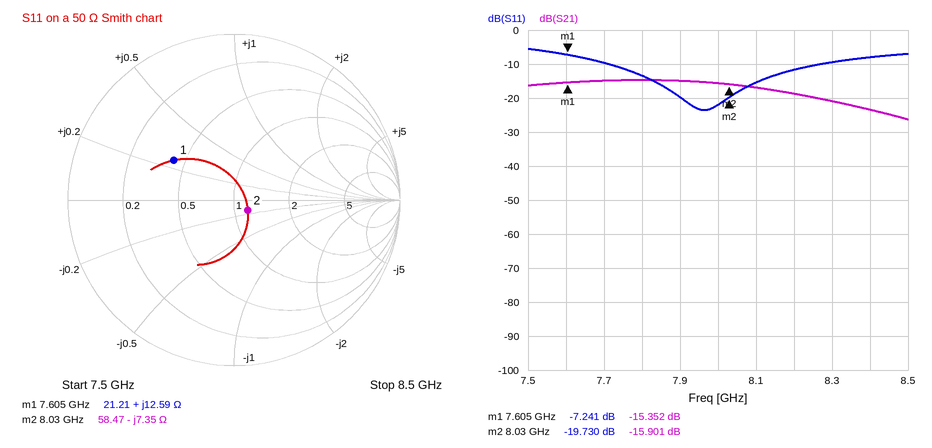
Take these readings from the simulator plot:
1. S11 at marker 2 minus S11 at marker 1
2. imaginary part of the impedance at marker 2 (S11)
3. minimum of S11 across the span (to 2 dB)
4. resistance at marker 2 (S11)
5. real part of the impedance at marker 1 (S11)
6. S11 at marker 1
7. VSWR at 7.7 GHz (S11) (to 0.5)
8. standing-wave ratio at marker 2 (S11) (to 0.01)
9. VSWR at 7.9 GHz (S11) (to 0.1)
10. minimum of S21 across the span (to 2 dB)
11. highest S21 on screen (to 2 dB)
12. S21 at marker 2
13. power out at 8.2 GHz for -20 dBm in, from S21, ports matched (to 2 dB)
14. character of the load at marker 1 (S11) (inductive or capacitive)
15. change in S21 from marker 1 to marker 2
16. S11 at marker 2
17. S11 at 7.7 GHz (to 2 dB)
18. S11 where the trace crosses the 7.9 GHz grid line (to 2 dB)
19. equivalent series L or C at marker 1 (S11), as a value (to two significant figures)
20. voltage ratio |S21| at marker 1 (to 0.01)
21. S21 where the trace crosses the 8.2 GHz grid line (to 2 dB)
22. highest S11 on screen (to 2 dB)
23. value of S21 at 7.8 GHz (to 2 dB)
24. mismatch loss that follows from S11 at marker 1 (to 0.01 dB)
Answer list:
-12.489 dB
-7.35 Ω
-24 dB
58.47 Ω
21.21 Ω
-7.241 dB
2.0
1.23
1.2
-26 dB
-14 dB
-15.901 dB
-38 dBm
inductive
-0.549 dB
-19.730 dB
-10 dB
-20 dB
260 pH
0.17
-18 dB
-6 dB
-14 dB
0.91 dB
